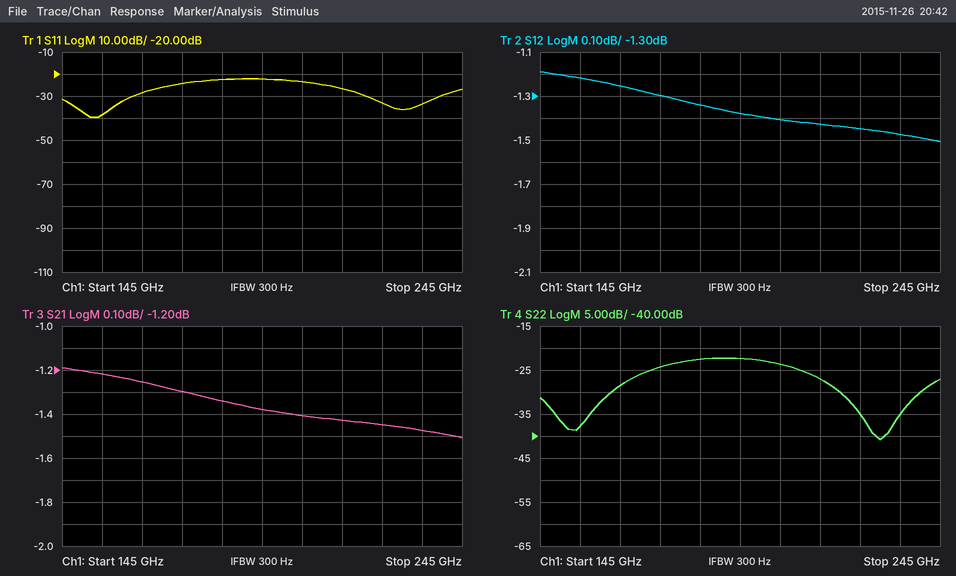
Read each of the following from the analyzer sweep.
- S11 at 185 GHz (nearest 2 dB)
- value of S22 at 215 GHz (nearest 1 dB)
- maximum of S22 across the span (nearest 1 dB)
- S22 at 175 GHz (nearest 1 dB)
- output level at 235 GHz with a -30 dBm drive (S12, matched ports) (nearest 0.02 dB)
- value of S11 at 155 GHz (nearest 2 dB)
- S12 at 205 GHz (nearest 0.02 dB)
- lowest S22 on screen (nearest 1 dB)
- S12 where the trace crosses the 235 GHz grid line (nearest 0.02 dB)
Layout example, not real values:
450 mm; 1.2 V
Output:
-22 dB; -27 dB; -22 dB; -24 dB; -31.48 dBm; -38 dB; -1.40 dB; -41 dB; -1.48 dB
